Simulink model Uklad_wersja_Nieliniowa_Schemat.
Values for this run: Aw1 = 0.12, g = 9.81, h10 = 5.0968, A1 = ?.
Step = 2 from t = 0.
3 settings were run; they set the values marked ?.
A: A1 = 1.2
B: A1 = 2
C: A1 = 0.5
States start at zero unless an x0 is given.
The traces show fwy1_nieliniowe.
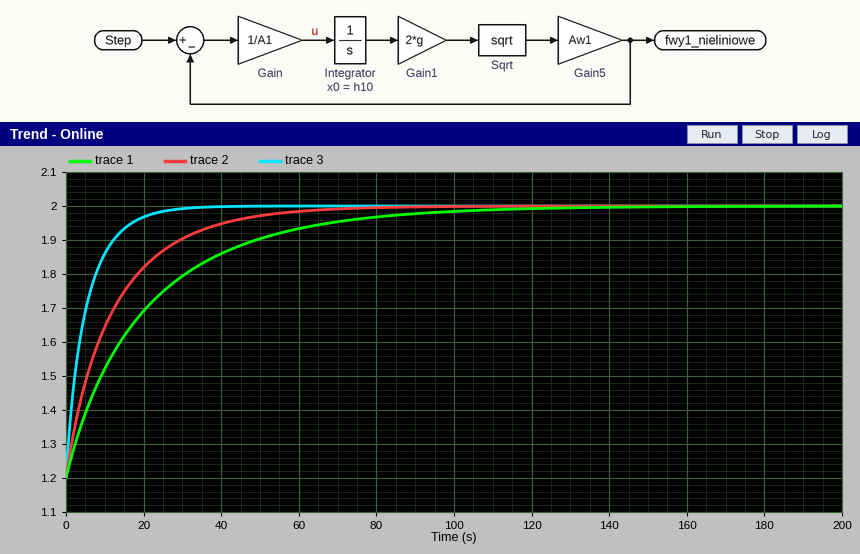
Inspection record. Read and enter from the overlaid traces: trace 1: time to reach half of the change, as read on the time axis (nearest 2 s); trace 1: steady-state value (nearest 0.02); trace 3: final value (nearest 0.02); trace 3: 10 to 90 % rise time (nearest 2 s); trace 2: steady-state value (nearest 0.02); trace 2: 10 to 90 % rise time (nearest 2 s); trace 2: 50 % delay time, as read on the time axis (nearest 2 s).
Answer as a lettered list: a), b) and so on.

a) 14 s
b) 2.00
c) 2.00
d) 14 s
e) 2.00
f) 32 s
g) 8 s
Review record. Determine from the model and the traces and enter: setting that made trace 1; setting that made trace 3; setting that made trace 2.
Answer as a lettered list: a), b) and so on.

a) B
b) C
c) A
